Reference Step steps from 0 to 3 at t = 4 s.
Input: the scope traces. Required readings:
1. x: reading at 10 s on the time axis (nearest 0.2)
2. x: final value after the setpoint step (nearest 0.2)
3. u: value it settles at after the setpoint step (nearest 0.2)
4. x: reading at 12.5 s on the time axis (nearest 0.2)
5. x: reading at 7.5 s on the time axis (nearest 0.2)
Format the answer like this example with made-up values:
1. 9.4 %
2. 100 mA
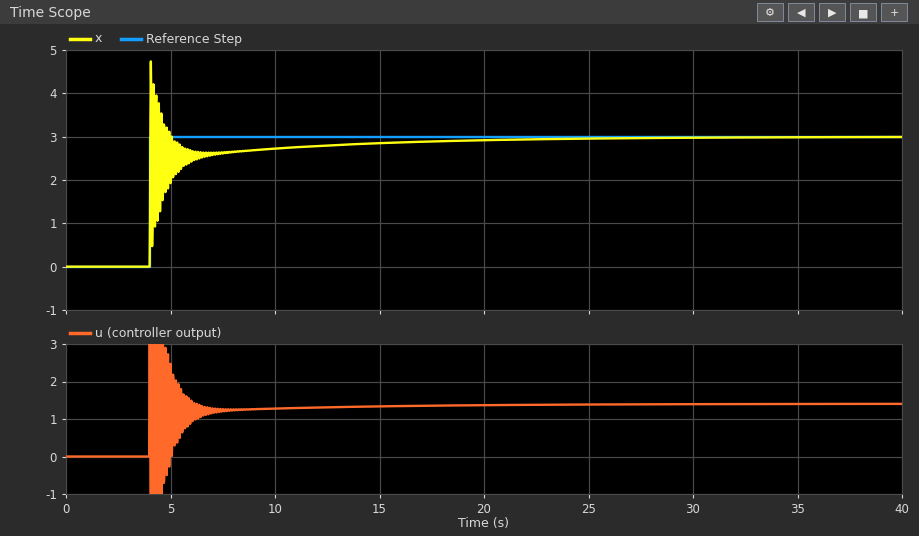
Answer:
1. 2.8
2. 3.0
3. 1.4
4. 2.8
5. 2.6
